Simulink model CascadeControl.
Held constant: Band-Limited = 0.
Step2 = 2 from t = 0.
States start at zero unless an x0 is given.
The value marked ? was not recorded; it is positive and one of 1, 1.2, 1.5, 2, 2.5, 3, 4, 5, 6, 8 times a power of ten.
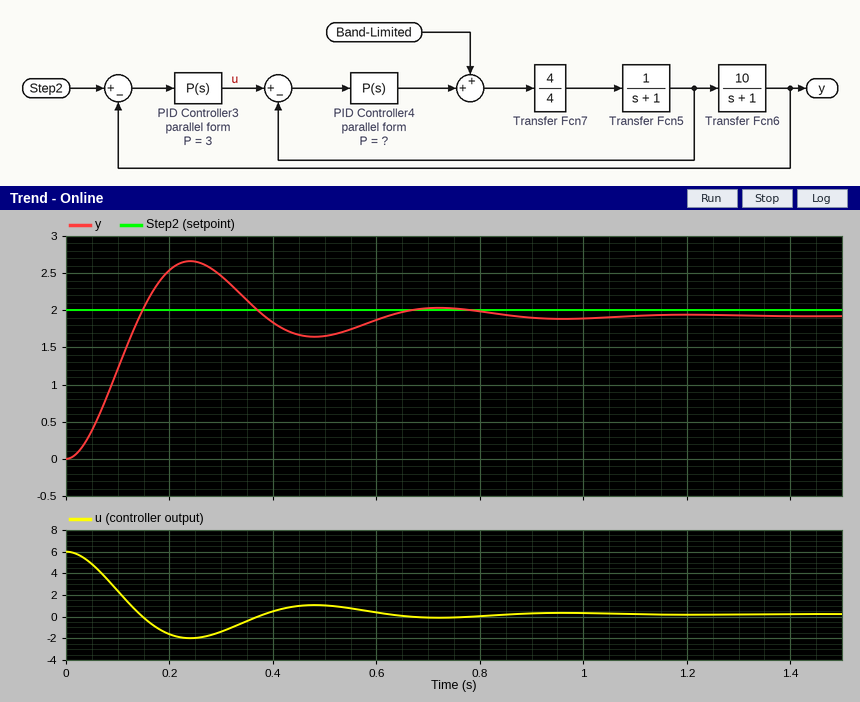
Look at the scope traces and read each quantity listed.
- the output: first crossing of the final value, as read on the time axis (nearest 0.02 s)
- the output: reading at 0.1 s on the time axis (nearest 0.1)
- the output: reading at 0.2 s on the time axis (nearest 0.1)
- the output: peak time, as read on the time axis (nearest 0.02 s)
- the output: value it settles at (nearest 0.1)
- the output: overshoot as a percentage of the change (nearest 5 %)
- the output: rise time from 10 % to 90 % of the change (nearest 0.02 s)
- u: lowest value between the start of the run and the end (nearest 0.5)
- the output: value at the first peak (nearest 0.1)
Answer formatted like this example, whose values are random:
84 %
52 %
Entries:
0.14 s
1.2
2.5
0.24 s
1.9
40 %
0.10 s
-2.0
2.7
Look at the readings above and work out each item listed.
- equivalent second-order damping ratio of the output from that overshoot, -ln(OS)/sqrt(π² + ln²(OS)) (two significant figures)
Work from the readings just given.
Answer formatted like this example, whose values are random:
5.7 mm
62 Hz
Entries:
0.28
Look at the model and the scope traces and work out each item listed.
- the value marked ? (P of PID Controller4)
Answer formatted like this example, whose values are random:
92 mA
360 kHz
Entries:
6
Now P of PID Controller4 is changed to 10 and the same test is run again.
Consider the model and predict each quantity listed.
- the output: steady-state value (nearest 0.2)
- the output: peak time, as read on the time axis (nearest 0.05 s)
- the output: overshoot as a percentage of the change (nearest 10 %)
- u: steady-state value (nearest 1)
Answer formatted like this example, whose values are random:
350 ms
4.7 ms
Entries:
2.0
0.20 s
30 %
0
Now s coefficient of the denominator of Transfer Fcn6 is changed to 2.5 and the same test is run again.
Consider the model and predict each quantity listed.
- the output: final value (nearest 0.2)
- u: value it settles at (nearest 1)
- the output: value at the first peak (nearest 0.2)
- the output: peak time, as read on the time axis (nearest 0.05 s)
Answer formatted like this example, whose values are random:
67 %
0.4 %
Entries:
2.0
0
2.4
0.40 s
